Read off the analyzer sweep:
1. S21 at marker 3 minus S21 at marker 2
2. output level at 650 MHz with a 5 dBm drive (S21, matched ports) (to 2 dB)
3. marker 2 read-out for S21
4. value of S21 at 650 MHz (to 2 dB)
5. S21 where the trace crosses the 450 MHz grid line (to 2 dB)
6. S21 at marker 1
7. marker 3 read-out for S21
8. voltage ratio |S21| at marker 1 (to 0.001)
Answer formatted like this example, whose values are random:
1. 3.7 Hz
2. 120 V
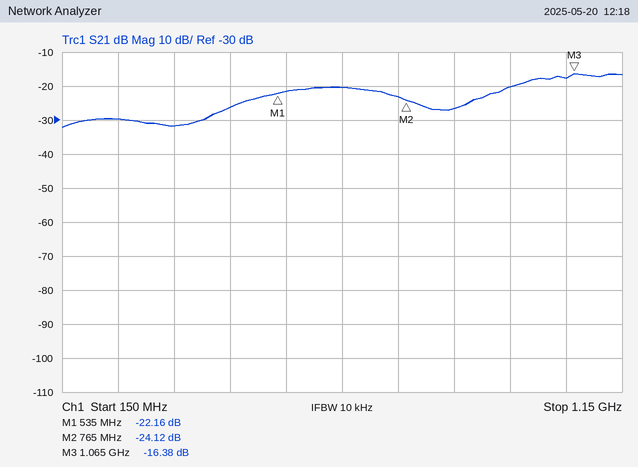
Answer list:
1. 7.74 dB
2. -16 dBm
3. -24.12 dB
4. -20 dB
5. -26 dB
6. -22.16 dB
7. -16.38 dB
8. 0.078
